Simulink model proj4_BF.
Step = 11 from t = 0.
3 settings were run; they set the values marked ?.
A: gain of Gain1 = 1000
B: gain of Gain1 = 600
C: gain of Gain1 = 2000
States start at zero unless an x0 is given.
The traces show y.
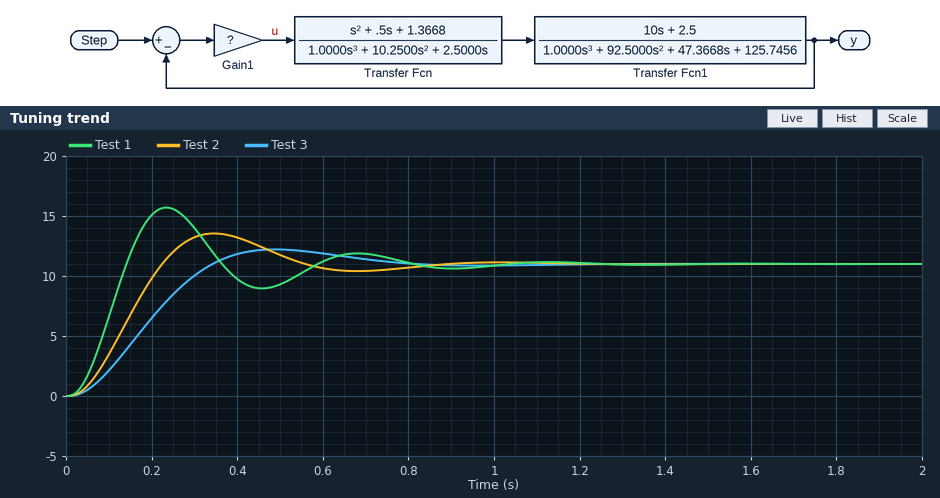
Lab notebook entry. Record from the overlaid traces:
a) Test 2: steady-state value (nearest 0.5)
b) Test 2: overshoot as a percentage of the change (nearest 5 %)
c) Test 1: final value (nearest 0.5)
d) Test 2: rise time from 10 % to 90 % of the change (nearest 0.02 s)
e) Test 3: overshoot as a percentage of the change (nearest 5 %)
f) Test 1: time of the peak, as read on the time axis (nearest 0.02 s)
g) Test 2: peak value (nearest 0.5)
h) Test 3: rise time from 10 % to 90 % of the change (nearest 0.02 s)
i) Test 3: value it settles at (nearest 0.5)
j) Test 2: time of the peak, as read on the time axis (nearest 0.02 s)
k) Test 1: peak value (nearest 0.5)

11.0
25 %
11.0
0.14 s
10 %
0.24 s
13.5
0.22 s
11.0
0.34 s
15.5
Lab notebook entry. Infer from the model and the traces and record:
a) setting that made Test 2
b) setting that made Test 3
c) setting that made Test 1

A
B
C
